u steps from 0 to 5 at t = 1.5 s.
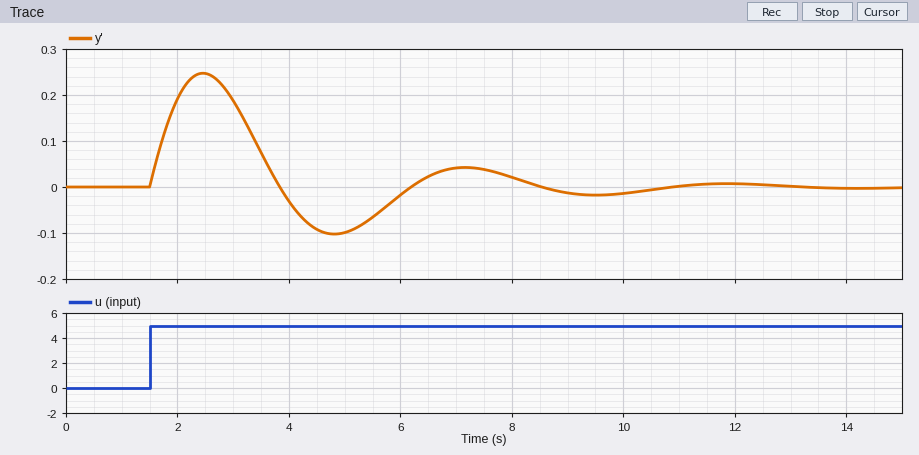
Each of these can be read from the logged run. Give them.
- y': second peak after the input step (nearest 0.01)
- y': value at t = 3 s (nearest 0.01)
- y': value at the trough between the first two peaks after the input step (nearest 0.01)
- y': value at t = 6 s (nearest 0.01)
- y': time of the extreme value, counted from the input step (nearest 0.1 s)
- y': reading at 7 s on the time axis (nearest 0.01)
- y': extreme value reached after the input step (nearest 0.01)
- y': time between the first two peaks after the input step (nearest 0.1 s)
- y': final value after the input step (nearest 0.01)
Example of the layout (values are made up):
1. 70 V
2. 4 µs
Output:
1. 0.04
2. 0.19
3. -0.10
4. -0.02
5. 1.0 s
6. 0.04
7. 0.25
8. 4.7 s
9. 0.00
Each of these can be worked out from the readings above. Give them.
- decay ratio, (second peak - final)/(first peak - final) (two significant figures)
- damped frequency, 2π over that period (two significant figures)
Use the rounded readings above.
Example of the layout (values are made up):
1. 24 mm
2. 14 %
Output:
1. 0.16
2. 1.3 rad/s
